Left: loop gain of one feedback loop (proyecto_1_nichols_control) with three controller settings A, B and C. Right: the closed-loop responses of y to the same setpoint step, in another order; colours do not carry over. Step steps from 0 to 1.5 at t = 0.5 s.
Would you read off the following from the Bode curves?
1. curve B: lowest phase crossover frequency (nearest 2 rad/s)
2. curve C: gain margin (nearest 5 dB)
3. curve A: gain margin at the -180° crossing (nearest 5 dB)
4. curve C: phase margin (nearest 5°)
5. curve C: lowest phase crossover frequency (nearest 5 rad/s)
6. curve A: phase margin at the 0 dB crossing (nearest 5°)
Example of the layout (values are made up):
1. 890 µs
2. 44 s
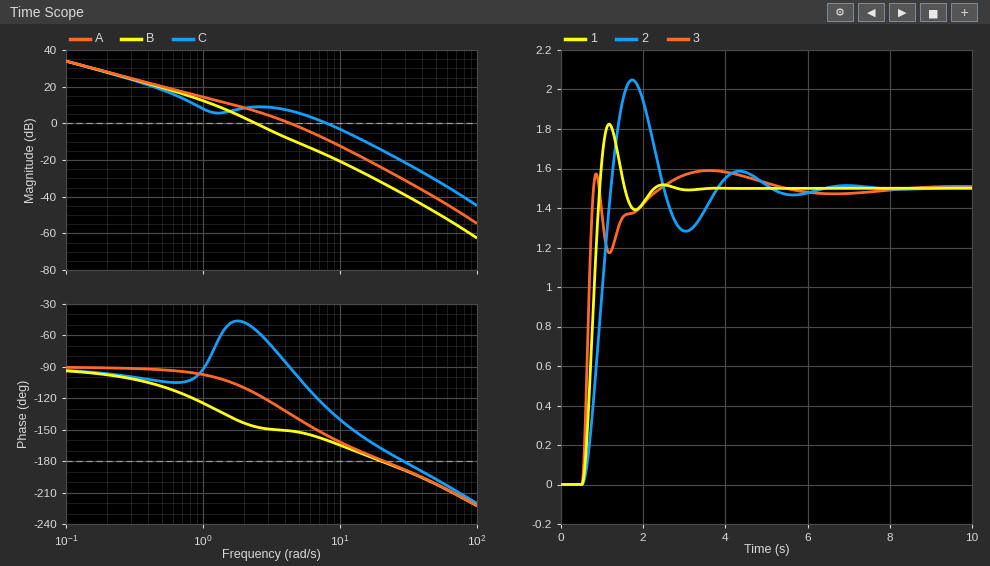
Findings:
1. 20 rad/s
2. 20 dB
3. 25 dB
4. 50°
5. 30 rad/s
6. 45°
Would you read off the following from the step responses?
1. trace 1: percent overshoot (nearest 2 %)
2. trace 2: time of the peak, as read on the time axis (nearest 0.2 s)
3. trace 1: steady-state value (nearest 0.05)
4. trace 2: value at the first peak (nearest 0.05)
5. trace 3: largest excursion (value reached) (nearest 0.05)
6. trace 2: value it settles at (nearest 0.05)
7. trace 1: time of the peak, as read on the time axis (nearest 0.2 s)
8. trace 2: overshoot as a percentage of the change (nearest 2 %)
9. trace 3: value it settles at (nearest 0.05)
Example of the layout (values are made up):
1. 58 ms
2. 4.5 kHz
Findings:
1. 22 %
2. 1.8 s
3. 1.50
4. 2.05
5. 1.60
6. 1.50
7. 1.2 s
8. 36 %
9. 1.50
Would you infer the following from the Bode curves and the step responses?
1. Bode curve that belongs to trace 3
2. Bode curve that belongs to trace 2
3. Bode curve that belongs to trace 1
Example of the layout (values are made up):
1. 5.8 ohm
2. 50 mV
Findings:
1. C
2. B
3. A
